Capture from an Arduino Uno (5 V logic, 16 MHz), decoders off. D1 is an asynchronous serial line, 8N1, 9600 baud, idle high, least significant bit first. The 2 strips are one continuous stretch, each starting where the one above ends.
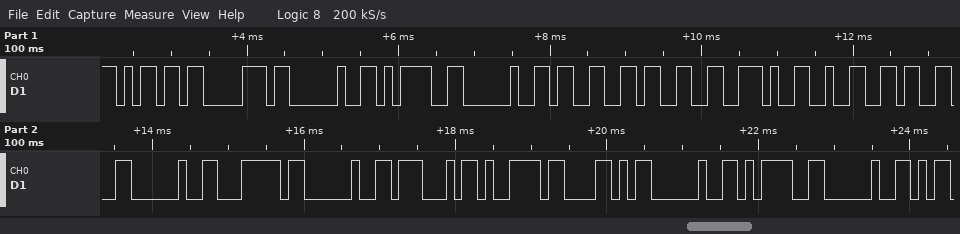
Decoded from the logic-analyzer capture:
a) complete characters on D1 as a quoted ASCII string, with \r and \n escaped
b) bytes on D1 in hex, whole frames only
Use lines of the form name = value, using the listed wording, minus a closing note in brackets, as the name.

complete characters on D1 as a quoted ASCII string, with \r and \n escaped = "mp = 33.23 | GyX = "
bytes on D1 in hex, whole frames only = 0x6D 0x70 0x20 0x3D 0x20 0x33 0x33 0x2E 0x32 0x33 0x20 0x7C 0x20 0x47 0x79 0x58 0x20 0x3D 0x20
